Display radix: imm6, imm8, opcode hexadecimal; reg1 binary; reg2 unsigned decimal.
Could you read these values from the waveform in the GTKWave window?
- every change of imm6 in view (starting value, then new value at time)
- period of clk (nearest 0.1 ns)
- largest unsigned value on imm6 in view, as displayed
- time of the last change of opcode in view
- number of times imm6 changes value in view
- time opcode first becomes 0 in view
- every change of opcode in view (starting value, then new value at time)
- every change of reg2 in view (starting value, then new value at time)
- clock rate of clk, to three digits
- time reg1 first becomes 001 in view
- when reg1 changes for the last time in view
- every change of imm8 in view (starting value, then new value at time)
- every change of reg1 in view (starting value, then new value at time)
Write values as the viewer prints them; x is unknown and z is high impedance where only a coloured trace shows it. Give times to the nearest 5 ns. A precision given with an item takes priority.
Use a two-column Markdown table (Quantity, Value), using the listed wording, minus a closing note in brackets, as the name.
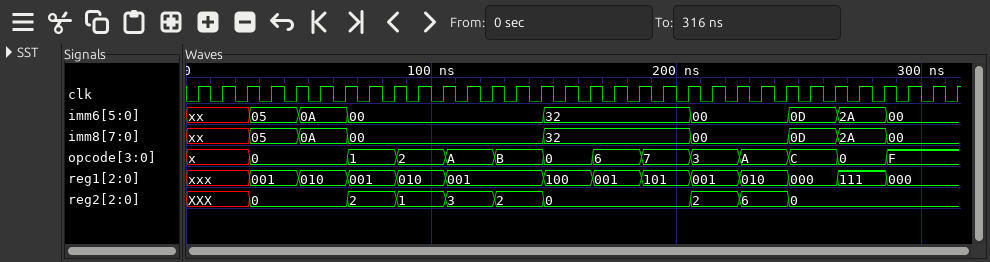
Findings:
| Quantity | Value |
|---|---|
| every change of imm6 in view | xx, 05 at 25 ns, 0A at 45 ns, 00 at 65 ns, 32 at 145 ns, 00 at 205 ns, 0D at 245 ns, 2A at 265 ns, 00 at 285 ns |
| period of clk | 10 ns |
| largest unsigned value on imm6 in view, as displayed | 32 |
| time of the last change of opcode in view | 285 ns |
| number of times imm6 changes value in view | 8 |
| time opcode first becomes 0 in view | 25 ns |
| every change of opcode in view | x, 0 at 25 ns, 1 at 65 ns, 2 at 85 ns, A at 105 ns, B at 125 ns, 0 at 145 ns, 6 at 165 ns, 7 at 185 ns, 3 at 205 ns, A at 225 ns, C at 245 ns, 0 at 265 ns, F at 285 ns |
| every change of reg2 in view | XXX, 0 at 25 ns, 2 at 65 ns, 1 at 85 ns, 3 at 105 ns, 2 at 125 ns, 0 at 145 ns, 2 at 205 ns, 6 at 225 ns, 0 at 245 ns |
| clock rate of clk, to three digits | 100 MHz |
| time reg1 first becomes 001 in view | 25 ns |
| when reg1 changes for the last time in view | 285 ns |
| every change of imm8 in view | xx, 05 at 25 ns, 0A at 45 ns, 00 at 65 ns, 32 at 145 ns, 00 at 205 ns, 0D at 245 ns, 2A at 265 ns, 00 at 285 ns |
| every change of reg1 in view | xxx, 001 at 25 ns, 010 at 45 ns, 001 at 65 ns, 010 at 85 ns, 001 at 105 ns, 100 at 145 ns, 001 at 165 ns, 101 at 185 ns, 001 at 205 ns, 010 at 225 ns, 000 at 245 ns, 111 at 265 ns, 000 at 285 ns |
